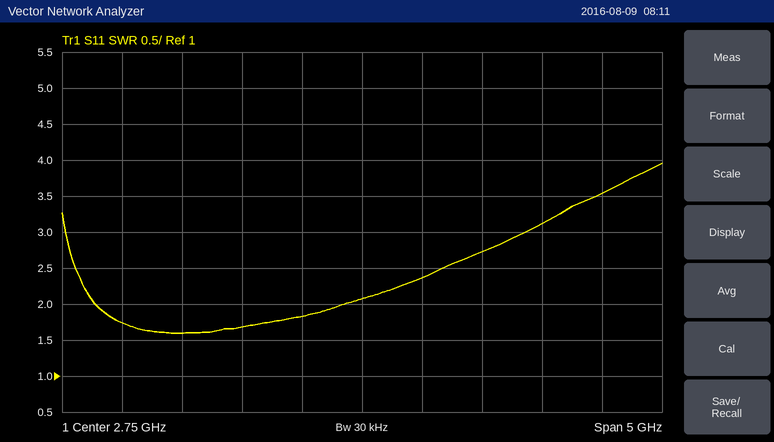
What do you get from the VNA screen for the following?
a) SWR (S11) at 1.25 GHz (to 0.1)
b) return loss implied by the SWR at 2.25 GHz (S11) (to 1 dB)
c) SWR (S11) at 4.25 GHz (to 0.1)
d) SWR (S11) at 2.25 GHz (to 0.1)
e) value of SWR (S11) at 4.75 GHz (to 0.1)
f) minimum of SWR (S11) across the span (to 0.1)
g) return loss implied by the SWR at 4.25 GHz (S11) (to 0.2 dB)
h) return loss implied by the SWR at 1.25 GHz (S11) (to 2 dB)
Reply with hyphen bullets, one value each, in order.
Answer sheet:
- 1.6
- 11 dB
- 3.1
- 1.8
- 3.5
- 1.6
- 5.8 dB
- 12 dB
